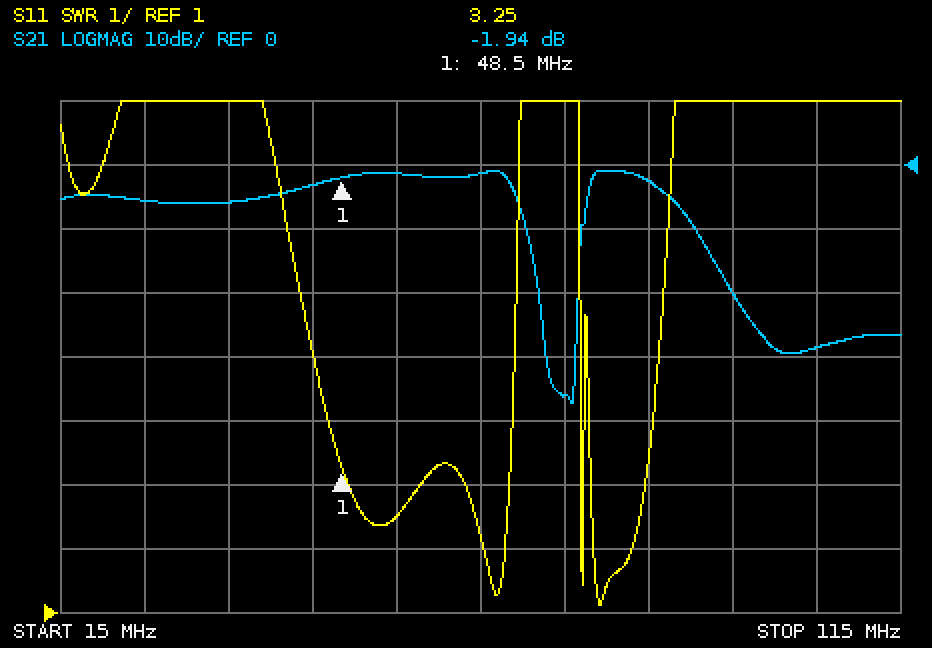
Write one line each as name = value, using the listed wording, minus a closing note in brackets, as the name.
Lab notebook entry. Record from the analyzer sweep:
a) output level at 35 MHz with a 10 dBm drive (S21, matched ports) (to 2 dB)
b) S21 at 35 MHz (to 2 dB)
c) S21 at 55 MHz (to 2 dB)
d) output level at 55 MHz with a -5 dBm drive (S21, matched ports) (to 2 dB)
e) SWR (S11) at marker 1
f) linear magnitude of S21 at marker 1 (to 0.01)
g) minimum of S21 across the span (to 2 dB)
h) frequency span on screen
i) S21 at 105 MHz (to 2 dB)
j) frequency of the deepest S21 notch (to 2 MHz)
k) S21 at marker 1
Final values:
output level at 35 MHz with a 10 dBm drive (S21, matched ports) = 4 dBm
S21 at 35 MHz = -6 dB
S21 at 55 MHz = -2 dB
output level at 55 MHz with a -5 dBm drive (S21, matched ports) = -6 dBm
SWR (S11) at marker 1 = 3.25
linear magnitude of S21 at marker 1 = 0.80
minimum of S21 across the span = -38 dB
frequency span on screen = 100 MHz
S21 at 105 MHz = -28 dB
frequency of the deepest S21 notch = 76 MHz
S21 at marker 1 = -1.94 dB
